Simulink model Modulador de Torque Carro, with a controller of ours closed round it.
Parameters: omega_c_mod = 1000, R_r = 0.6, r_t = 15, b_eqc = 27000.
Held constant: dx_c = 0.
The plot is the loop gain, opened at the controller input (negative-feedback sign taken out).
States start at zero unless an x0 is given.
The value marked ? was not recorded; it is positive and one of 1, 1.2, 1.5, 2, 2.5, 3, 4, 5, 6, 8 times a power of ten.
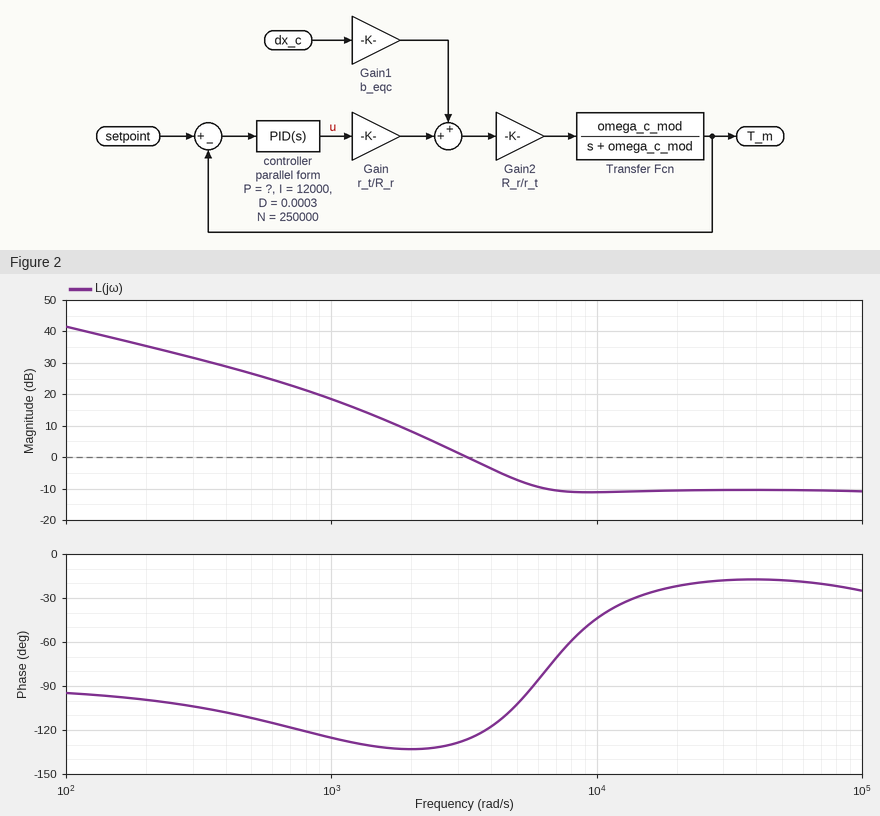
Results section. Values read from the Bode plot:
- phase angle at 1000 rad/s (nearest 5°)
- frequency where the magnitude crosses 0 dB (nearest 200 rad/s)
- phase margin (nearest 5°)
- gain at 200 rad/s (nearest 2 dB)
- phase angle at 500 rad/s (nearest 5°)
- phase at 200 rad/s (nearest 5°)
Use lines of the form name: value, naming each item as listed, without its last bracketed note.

phase angle at 1000 rad/s: -125°
frequency where the magnitude crosses 0 dB: 3200 rad/s
phase margin: 55°
gain at 200 rad/s: 36 dB
phase angle at 500 rad/s: -110°
phase at 200 rad/s: -100°
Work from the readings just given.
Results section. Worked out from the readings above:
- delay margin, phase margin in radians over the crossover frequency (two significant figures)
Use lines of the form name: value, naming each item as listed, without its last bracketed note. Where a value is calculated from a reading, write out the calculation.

delay margin, phase margin in radians over the crossover frequency: 55 × π / 180 / 3200 = 0.00030 s
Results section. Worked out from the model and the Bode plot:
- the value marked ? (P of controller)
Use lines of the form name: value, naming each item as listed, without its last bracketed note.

the value marked ?: 2
